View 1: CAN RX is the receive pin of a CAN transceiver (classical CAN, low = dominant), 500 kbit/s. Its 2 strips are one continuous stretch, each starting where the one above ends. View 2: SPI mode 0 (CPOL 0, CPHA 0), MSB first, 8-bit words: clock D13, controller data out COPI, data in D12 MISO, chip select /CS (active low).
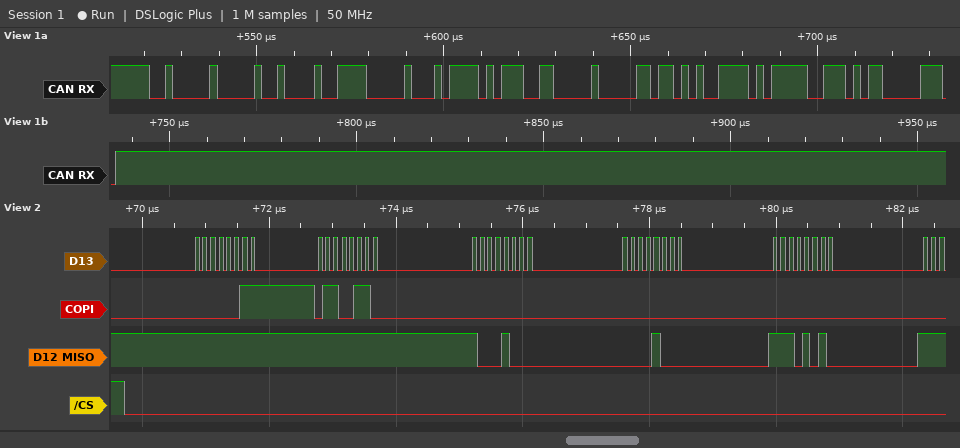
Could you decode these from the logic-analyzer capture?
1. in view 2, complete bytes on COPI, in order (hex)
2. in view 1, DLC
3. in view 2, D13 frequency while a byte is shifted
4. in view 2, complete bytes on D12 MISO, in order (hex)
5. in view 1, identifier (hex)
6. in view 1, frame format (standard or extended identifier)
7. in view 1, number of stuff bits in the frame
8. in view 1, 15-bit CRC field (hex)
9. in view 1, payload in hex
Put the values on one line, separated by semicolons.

0x03 0x66 0x00 0x00 0x00; 8; 8 MHz; 0xFF 0xFF 0x88 0x08 0xEA; 0x200; standard; 7; 0x3AC1; 4F 00 BD 73 00 2D 4F 5F
